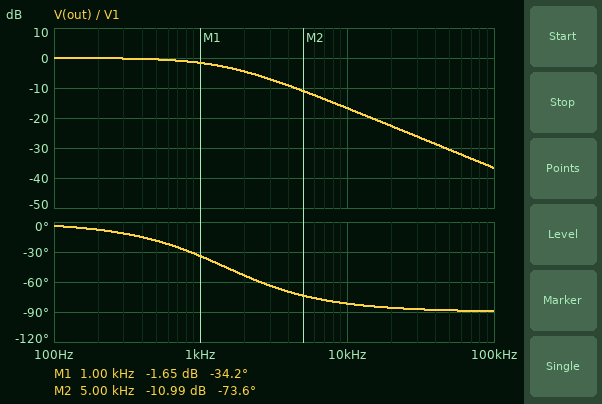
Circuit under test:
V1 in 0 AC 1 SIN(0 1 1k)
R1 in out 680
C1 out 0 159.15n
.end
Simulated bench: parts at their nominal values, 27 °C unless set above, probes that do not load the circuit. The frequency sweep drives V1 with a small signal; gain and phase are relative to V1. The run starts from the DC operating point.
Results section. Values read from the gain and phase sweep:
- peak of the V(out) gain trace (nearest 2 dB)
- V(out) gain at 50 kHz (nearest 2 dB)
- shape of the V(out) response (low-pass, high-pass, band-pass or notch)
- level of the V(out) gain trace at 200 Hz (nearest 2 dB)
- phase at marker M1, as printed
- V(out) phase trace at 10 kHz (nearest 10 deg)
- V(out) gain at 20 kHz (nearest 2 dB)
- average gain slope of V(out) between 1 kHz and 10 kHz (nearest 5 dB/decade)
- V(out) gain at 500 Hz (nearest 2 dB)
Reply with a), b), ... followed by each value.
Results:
a) 0 dB
b) -30 dB
c) low-pass
d) 0 dB
e) -34.2 deg
f) -80 deg
g) -22 dB
h) -15 dB/decade
i) 0 dB
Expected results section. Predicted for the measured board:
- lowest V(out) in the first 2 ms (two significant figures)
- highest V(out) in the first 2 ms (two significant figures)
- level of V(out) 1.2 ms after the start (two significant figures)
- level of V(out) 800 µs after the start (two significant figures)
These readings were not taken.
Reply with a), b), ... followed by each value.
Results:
a) -830 mV
b) 850 mV
c) 510 mV
d) -790 mV
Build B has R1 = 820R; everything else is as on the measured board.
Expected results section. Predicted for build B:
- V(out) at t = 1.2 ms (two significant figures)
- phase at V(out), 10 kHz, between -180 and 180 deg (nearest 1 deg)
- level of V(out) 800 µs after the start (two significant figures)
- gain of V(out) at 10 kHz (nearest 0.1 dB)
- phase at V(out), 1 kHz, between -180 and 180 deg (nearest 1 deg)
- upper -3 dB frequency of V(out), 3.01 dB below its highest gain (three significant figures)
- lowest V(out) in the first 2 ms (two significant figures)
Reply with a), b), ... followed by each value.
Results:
a) 420 mV
b) -83 deg
c) -720 mV
d) -18.3 dB
e) -39 deg
f) 1.22 kHz
g) -770 mV
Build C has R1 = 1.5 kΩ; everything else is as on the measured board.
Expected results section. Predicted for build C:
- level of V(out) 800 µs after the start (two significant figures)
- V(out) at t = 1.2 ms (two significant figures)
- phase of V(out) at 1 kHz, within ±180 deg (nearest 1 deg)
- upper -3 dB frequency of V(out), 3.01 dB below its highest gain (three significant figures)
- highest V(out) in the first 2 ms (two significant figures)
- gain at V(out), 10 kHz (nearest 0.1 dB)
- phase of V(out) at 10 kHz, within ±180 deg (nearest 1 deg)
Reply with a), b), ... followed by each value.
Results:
a) -420 mV
b) 150 mV
c) -56 deg
d) 667 Hz
e) 640 mV
f) -23.5 dB
g) -86 deg
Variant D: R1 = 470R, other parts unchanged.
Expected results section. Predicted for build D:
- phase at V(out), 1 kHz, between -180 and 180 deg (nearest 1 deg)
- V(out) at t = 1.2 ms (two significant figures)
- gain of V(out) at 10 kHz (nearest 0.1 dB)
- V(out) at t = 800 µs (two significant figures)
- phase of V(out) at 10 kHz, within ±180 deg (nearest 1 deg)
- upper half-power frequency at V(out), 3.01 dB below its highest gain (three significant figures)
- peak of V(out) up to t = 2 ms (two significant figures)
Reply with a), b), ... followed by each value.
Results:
a) -25 deg
b) 660 mV
c) -13.6 dB
d) -900 mV
e) -78 deg
f) 2.13 kHz
g) 910 mV
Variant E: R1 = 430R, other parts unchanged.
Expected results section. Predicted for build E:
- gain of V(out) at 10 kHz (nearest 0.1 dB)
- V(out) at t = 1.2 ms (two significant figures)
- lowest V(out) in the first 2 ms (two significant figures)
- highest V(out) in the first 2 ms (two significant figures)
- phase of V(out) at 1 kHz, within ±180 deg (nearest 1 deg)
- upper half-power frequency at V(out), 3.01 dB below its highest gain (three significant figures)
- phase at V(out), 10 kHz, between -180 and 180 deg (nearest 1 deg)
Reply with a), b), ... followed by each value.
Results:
a) -12.9 dB
b) 690 mV
c) -920 mV
d) 920 mV
e) -23 deg
f) 2.33 kHz
g) -77 deg
